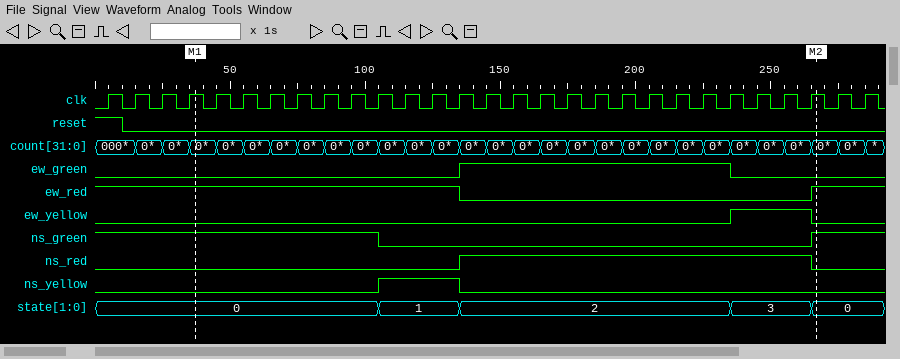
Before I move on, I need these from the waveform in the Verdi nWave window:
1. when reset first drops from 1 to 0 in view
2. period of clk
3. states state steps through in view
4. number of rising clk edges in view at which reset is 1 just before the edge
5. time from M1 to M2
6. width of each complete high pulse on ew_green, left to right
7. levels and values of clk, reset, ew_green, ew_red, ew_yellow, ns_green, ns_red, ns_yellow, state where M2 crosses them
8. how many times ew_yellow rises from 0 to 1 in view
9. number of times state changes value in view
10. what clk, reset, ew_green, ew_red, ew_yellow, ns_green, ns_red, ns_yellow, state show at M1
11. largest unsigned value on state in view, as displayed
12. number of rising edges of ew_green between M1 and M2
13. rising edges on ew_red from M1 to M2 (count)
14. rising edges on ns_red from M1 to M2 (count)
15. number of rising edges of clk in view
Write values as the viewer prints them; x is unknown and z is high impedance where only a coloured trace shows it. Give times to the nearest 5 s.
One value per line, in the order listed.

10 s
10 s
0, 1, 2, 3, 0
1
230 s
100 s
clk=1, reset=0, ew_green=0, ew_red=1, ew_yellow=0, ns_green=1, ns_red=0, ns_yellow=0, state=0
1
4
clk=1, reset=0, ew_green=0, ew_red=1, ew_yellow=0, ns_green=1, ns_red=0, ns_yellow=0, state=0
3
1
1
1
29
